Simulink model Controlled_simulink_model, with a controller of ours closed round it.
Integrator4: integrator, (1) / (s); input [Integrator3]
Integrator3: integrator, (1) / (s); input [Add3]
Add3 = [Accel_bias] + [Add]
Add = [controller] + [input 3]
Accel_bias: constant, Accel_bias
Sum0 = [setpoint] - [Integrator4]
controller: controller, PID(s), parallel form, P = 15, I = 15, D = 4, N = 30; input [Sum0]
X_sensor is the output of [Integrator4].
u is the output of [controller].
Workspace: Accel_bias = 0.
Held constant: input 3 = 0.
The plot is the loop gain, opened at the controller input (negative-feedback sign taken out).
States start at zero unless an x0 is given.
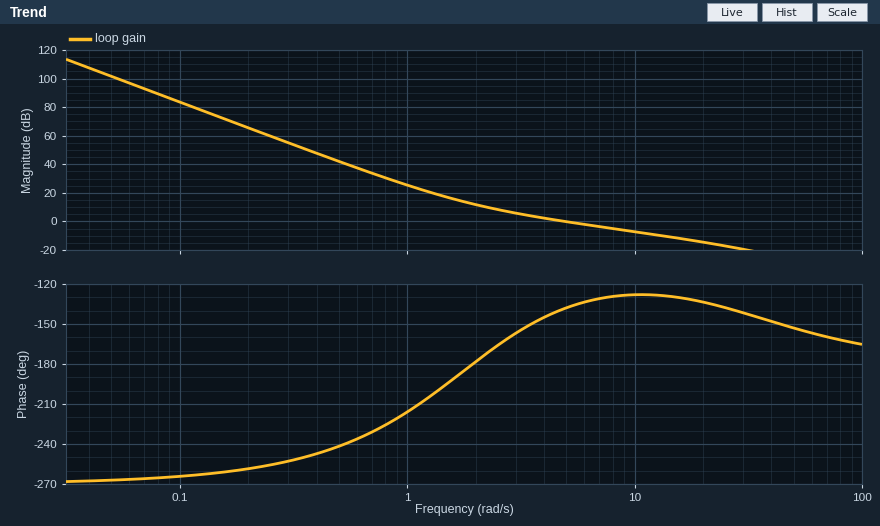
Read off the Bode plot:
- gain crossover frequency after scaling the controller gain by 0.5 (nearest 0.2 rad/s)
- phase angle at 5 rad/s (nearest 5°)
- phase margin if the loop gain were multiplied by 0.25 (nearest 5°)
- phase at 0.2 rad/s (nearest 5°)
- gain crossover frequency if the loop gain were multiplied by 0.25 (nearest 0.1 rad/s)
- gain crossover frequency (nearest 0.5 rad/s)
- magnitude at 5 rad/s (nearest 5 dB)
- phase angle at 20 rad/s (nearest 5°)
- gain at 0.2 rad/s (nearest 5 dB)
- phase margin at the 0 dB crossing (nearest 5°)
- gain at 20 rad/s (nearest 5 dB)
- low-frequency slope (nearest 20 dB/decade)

3.0 rad/s
-140°
0°
-260°
2.0 rad/s
5.0 rad/s
0 dB
-135°
65 dB
40°
-15 dB
-60 dB/decade
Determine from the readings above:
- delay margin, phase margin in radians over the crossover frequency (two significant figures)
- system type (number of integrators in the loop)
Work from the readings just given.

0.14 s
3
